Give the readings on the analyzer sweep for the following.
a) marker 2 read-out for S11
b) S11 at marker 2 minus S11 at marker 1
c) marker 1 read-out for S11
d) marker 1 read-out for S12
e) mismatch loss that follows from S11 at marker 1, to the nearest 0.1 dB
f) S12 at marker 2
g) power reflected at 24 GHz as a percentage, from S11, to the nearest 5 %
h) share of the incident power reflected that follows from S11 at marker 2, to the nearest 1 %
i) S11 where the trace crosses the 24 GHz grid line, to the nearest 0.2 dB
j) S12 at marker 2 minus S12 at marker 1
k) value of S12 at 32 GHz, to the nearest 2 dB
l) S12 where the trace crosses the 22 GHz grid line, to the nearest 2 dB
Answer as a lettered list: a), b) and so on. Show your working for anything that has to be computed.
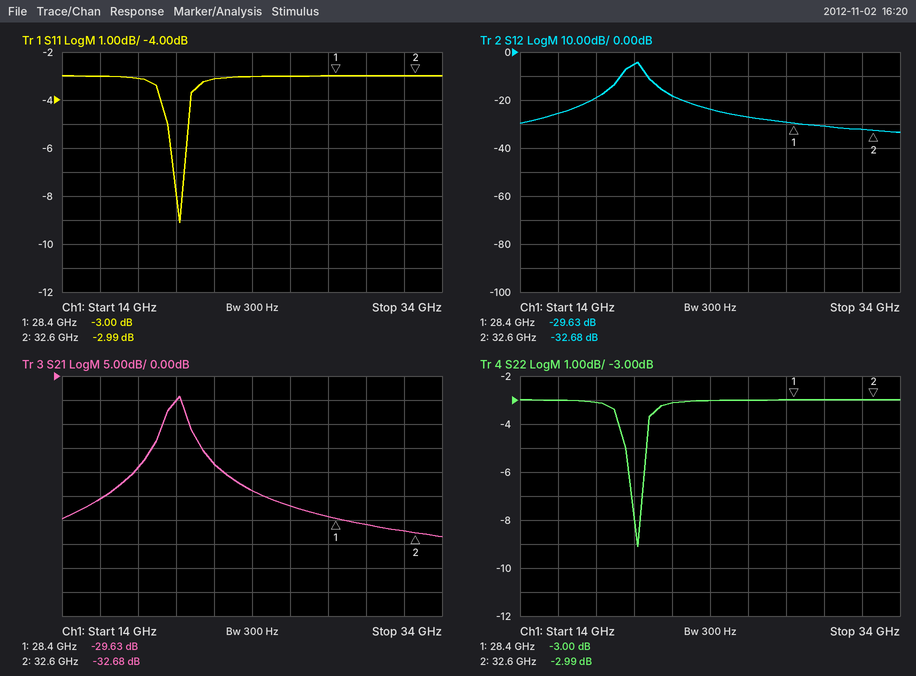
a) -2.99 dB
b) -2.99 − (-3) = 0.01 dB
c) -3.00 dB
d) -29.63 dB
e) −10 log10(1 − 10^(-3/10)) ≈ 3.0 dB
f) -32.68 dB
g) 10^(-3/10) ≈ 50 %
h) 10^(-2.99/10) ≈ 50 %
i) -3.0 dB
j) -32.68 − (-29.63) = -3.05 dB
k) -32 dB
l) -18 dB
